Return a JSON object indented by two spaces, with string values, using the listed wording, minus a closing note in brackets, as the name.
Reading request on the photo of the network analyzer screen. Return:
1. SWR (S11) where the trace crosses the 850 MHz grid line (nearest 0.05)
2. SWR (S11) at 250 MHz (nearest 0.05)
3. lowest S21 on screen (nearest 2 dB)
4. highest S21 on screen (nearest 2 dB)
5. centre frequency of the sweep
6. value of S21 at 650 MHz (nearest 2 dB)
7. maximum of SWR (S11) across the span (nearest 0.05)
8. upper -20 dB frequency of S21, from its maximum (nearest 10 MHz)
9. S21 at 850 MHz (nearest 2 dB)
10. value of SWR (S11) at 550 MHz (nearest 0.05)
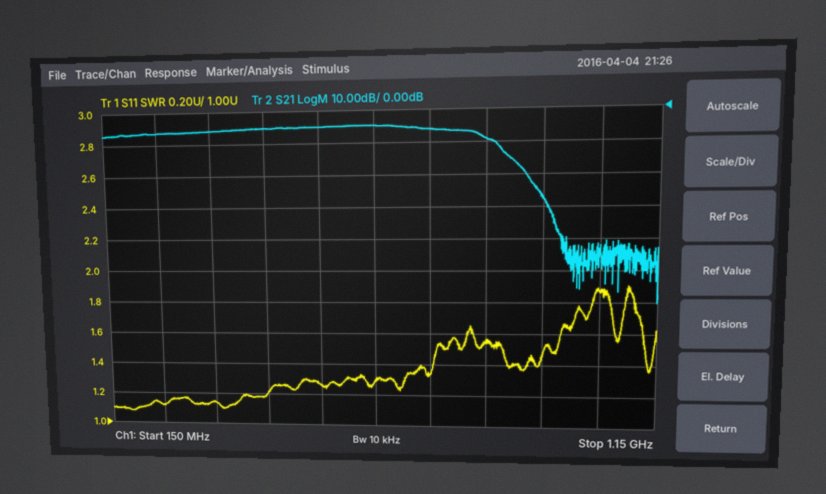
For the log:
{
  "SWR (S11) where the trace crosses the 850 MHz grid line": "1.55",
  "SWR (S11) at 250 MHz": "1.10",
  "lowest S21 on screen": "-60 dB",
  "highest S21 on screen": "-4 dB",
  "centre frequency of the sweep": "650 MHz",
  "value of S21 at 650 MHz": "-4 dB",
  "maximum of SWR (S11) across the span": "1.90",
  "upper -20 dB frequency of S21, from its maximum": "940 MHz",
  "S21 at 850 MHz": "-10 dB",
  "value of SWR (S11) at 550 MHz": "1.25"
}
